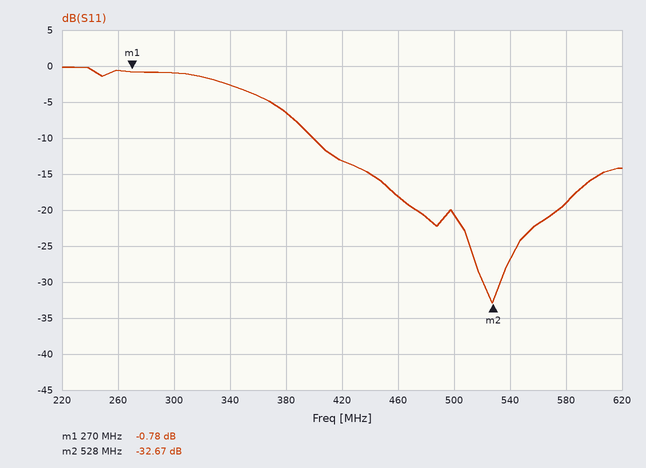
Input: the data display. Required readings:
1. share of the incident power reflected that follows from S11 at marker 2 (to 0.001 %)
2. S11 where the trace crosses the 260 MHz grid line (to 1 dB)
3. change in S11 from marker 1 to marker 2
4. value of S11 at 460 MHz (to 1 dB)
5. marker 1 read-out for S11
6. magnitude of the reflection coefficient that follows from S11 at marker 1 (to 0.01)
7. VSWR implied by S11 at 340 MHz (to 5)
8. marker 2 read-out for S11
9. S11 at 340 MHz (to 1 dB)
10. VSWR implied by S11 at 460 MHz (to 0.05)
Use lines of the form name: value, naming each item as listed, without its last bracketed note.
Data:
share of the incident power reflected that follows from S11 at marker 2: 0.054 %
S11 where the trace crosses the 260 MHz grid line: -1 dB
change in S11 from marker 1 to marker 2: -31.89 dB
value of S11 at 460 MHz: -18 dB
marker 1 read-out for S11: -0.78 dB
magnitude of the reflection coefficient that follows from S11 at marker 1: 0.91
VSWR implied by S11 at 340 MHz: 5
marker 2 read-out for S11: -32.67 dB
S11 at 340 MHz: -3 dB
VSWR implied by S11 at 460 MHz: 1.30
